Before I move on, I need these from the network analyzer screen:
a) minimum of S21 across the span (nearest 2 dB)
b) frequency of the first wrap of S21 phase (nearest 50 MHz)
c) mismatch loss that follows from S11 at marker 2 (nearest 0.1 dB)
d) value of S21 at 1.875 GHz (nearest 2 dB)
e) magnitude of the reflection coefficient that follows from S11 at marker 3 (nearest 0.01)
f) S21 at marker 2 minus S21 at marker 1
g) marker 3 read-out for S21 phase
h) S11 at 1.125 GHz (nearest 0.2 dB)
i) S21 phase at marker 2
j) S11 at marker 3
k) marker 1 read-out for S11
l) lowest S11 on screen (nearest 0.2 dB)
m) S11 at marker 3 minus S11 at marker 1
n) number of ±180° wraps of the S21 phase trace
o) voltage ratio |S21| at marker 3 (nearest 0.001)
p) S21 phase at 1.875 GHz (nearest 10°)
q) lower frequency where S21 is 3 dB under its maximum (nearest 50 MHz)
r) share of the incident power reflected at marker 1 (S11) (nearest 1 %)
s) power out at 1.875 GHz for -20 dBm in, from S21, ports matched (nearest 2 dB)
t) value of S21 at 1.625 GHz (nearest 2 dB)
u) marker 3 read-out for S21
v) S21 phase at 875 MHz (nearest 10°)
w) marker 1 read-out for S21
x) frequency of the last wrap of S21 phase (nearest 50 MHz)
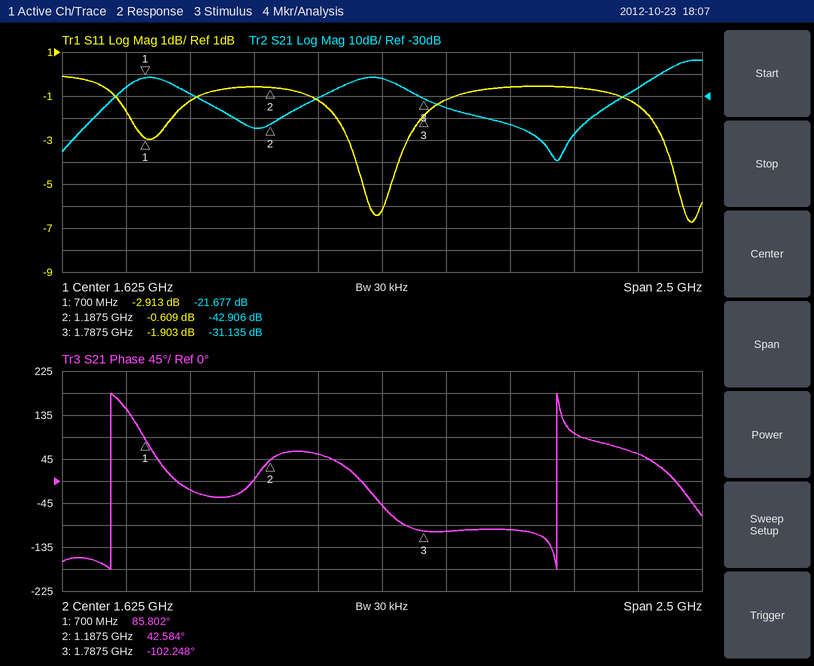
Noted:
-60 dB
550 MHz
8.8 dB
-36 dB
0.80
-21.229 dB
-102.248°
-0.6 dB
42.584°
-1.903 dB
-2.913 dB
-6.8 dB
1.010 dB
2
0.028
-100°
2.75 GHz
51 %
-56 dBm
-22 dB
-31.135 dB
-20°
-21.677 dB
2.30 GHz
